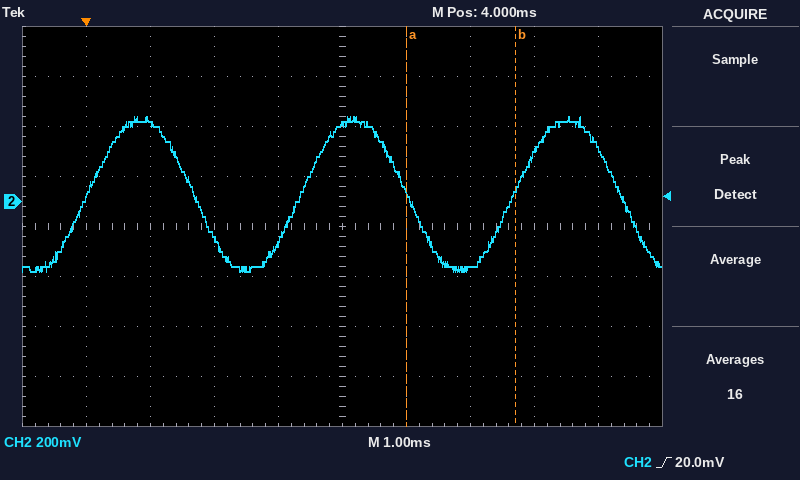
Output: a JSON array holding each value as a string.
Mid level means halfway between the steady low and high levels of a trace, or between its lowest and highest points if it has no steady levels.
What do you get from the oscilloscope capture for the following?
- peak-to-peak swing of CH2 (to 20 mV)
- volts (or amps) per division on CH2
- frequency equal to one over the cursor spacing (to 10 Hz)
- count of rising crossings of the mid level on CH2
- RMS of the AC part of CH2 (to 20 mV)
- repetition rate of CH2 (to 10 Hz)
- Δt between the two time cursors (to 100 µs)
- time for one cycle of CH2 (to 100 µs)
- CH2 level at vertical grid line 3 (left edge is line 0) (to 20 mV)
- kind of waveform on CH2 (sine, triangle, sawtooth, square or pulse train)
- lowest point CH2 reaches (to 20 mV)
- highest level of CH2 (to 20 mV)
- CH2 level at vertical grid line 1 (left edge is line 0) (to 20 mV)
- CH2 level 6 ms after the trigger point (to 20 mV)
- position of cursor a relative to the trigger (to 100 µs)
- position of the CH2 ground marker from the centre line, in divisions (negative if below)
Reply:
["620 mV", "200 mV", "590 Hz", "3", "220 mV", "300 Hz", "1.7 ms", "3.3 ms", "-140 mV", "sine", "-280 mV", "340 mV", "20 mV", "-260 mV", "+5.0 ms", "+0.5 div"]
